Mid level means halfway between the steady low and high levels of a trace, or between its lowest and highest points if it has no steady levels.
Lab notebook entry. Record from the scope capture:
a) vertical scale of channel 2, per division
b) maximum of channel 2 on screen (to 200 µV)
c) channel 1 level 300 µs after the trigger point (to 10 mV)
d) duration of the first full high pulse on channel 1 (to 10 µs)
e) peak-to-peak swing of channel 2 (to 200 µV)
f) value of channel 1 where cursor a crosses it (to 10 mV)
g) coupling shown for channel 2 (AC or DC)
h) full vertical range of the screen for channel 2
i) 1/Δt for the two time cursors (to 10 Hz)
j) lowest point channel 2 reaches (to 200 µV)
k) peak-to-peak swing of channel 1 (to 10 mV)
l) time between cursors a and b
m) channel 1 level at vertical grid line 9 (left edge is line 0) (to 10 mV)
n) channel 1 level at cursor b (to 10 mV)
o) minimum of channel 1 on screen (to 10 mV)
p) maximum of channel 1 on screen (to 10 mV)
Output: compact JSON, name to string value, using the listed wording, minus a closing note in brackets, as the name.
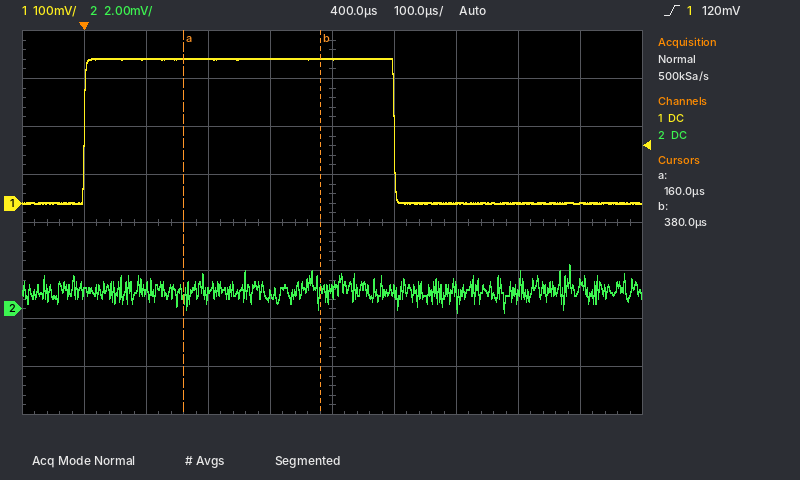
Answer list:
{"vertical scale of channel 2, per division": "2 mV", "maximum of channel 2 on screen": "1.8 mV", "channel 1 level 300 µs after the trigger point": "300 mV", "duration of the first full high pulse on channel 1": "500 µs", "peak-to-peak swing of channel 2": "2.0 mV", "value of channel 1 where cursor a crosses it": "300 mV", "coupling shown for channel 2": "DC", "full vertical range of the screen for channel 2": "16 mV", "1/Δt for the two time cursors": "4.55 kHz", "lowest point channel 2 reaches": "-200 µV", "peak-to-peak swing of channel 1": "300 mV", "time between cursors a and b": "220 µs", "channel 1 level at vertical grid line 9 (left edge is line 0)": "0 mV", "channel 1 level at cursor b": "300 mV", "minimum of channel 1 on screen": "0 mV", "maximum of channel 1 on screen": "300 mV"}
